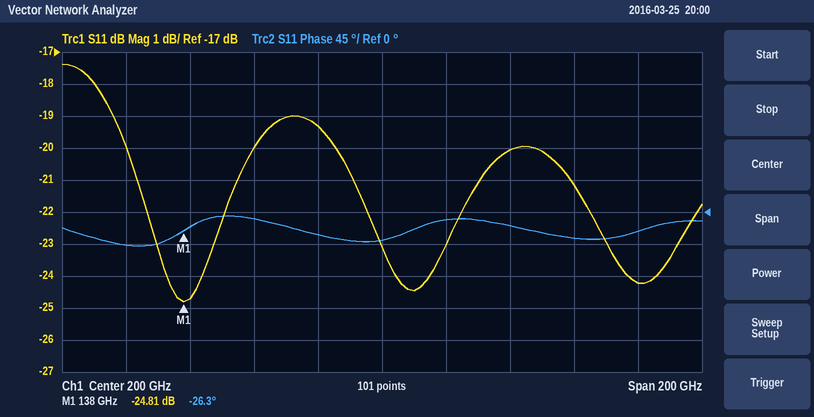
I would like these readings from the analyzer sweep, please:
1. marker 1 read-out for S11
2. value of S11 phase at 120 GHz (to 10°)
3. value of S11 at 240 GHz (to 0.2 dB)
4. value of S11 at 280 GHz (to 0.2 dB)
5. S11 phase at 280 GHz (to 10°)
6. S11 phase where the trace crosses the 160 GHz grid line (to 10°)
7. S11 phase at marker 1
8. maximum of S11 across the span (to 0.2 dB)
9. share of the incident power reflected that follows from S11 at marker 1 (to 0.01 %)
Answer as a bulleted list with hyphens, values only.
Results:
- -24.81 dB
- -50°
- -20.0 dB
- -24.2 dB
- -30°
- -10°
- -26.3°
- -17.4 dB
- 0.33 %
